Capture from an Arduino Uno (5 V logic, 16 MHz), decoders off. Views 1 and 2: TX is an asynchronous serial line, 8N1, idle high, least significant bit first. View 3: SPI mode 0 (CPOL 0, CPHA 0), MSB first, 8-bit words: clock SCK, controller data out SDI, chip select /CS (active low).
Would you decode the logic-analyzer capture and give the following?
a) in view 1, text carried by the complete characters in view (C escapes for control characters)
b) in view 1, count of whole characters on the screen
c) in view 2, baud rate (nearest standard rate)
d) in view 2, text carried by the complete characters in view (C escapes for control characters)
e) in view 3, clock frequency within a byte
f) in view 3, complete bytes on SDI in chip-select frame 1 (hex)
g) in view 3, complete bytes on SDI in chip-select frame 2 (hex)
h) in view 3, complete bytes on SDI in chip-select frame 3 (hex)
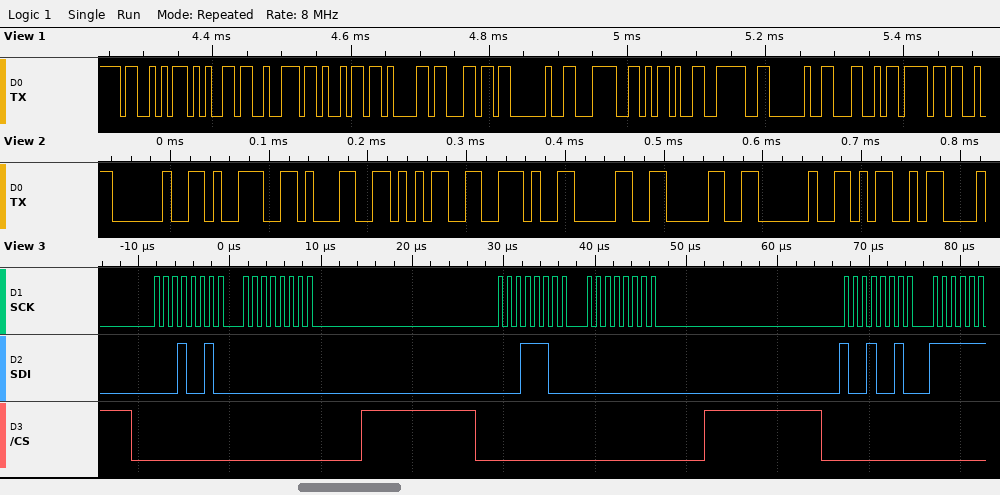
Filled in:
"Serial <-> Lo"
13
115200 baud
" 915.00 M"
1 MHz
12 00
1C 00
92
